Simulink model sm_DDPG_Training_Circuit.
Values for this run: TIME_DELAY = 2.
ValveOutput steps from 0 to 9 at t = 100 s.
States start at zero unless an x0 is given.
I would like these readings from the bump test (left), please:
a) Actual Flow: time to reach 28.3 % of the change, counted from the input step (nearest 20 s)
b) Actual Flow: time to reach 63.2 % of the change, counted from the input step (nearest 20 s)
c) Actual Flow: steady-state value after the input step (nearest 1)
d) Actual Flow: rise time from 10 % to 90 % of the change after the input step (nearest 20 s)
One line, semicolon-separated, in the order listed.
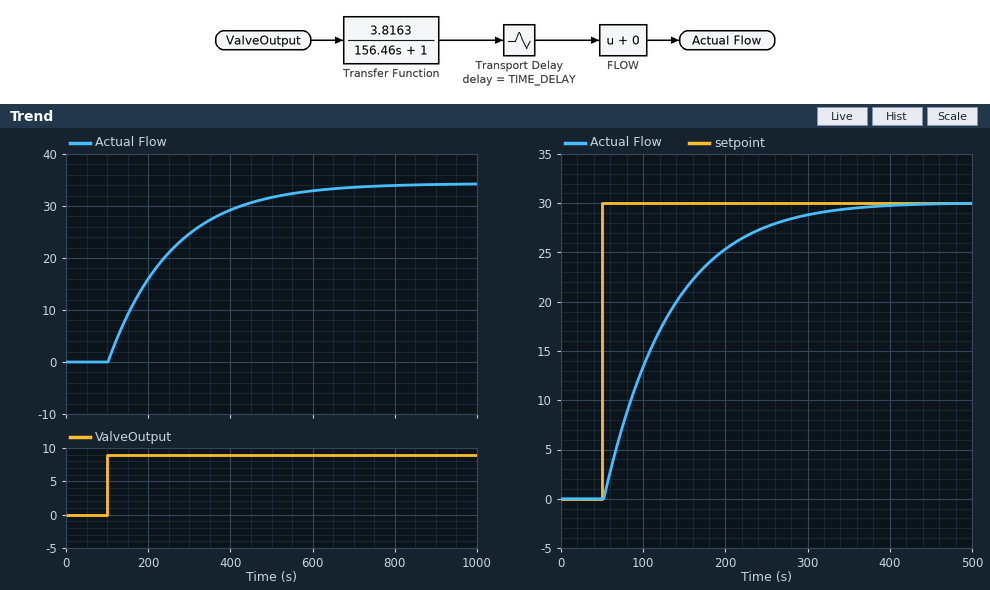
60 s; 160 s; 34; 340 s
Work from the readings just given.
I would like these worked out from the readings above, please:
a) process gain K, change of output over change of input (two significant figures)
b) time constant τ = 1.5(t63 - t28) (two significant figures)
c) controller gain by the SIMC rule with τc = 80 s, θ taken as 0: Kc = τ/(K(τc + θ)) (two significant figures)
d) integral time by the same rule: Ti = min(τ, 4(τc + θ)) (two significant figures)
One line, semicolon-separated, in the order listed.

3.8; 150 s; 0.49; 150 s
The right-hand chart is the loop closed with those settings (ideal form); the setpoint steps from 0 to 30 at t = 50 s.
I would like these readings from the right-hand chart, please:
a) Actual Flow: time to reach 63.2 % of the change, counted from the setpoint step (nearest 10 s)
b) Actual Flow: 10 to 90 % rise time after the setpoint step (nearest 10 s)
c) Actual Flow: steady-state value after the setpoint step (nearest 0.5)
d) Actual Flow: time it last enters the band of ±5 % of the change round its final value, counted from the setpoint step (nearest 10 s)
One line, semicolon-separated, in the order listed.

80 s; 170 s; 30.0; 230 s
